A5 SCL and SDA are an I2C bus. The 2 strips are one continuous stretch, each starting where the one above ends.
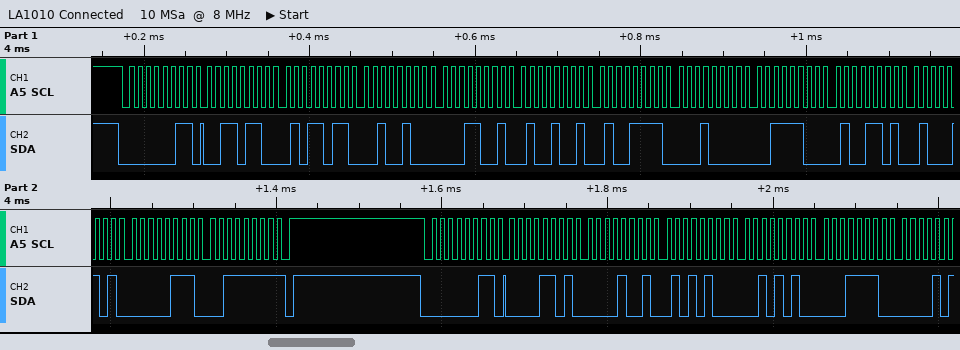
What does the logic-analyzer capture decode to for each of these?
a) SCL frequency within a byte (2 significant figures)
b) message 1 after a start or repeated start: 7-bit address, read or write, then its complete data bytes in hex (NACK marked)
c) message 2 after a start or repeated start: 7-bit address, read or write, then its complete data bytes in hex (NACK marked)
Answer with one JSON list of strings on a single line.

["100 kHz", "0x01 read: 36 5B 24 19 49 4F 10 3C 4D 45 07 3F NACK", "0x01 read: 0D 09 54 2A 1E"]
